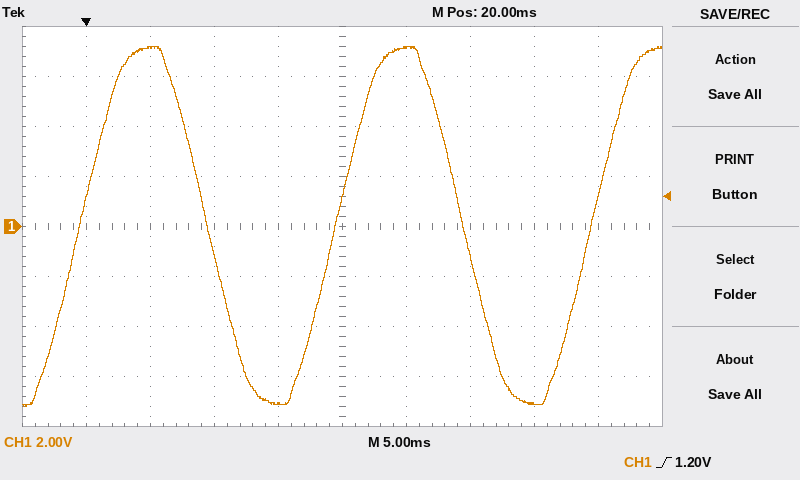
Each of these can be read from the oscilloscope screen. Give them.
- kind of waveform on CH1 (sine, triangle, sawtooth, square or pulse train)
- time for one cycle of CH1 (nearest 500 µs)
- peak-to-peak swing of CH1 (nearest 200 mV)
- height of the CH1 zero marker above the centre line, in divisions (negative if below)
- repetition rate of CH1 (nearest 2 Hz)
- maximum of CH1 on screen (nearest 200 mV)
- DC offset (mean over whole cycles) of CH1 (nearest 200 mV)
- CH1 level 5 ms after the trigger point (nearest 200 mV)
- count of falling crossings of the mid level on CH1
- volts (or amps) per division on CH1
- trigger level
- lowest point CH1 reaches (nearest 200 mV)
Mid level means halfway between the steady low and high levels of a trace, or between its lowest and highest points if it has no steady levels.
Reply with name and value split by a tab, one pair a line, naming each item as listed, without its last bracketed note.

kind of waveform on CH1	sine
time for one cycle of CH1	20.0 ms
peak-to-peak swing of CH1	14.4 V
height of the CH1 zero marker above the centre line, in divisions	0.0 div
repetition rate of CH1	50 Hz
maximum of CH1 on screen	7.2 V
DC offset (mean over whole cycles) of CH1	0.0 V
CH1 level 5 ms after the trigger point	7.2 V
count of falling crossings of the mid level on CH1	2
volts (or amps) per division on CH1	2 V
trigger level	1.20 V
lowest point CH1 reaches	-7.2 V
